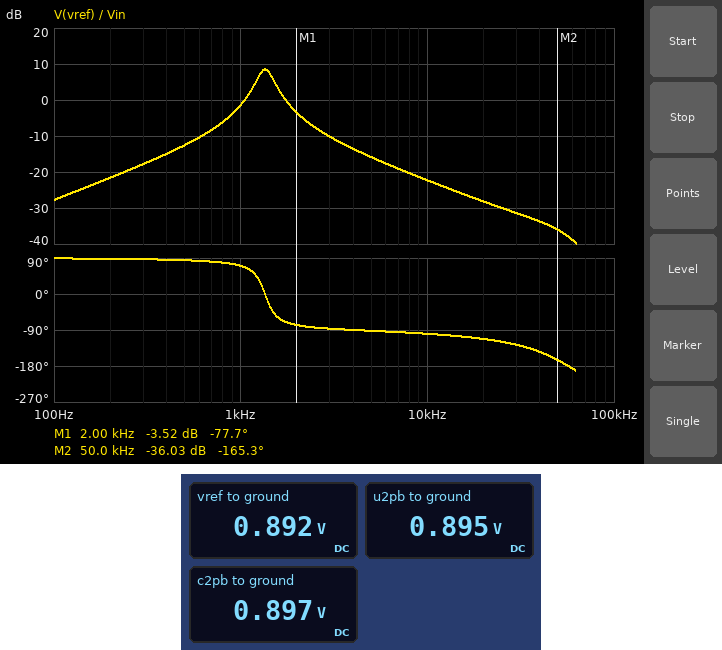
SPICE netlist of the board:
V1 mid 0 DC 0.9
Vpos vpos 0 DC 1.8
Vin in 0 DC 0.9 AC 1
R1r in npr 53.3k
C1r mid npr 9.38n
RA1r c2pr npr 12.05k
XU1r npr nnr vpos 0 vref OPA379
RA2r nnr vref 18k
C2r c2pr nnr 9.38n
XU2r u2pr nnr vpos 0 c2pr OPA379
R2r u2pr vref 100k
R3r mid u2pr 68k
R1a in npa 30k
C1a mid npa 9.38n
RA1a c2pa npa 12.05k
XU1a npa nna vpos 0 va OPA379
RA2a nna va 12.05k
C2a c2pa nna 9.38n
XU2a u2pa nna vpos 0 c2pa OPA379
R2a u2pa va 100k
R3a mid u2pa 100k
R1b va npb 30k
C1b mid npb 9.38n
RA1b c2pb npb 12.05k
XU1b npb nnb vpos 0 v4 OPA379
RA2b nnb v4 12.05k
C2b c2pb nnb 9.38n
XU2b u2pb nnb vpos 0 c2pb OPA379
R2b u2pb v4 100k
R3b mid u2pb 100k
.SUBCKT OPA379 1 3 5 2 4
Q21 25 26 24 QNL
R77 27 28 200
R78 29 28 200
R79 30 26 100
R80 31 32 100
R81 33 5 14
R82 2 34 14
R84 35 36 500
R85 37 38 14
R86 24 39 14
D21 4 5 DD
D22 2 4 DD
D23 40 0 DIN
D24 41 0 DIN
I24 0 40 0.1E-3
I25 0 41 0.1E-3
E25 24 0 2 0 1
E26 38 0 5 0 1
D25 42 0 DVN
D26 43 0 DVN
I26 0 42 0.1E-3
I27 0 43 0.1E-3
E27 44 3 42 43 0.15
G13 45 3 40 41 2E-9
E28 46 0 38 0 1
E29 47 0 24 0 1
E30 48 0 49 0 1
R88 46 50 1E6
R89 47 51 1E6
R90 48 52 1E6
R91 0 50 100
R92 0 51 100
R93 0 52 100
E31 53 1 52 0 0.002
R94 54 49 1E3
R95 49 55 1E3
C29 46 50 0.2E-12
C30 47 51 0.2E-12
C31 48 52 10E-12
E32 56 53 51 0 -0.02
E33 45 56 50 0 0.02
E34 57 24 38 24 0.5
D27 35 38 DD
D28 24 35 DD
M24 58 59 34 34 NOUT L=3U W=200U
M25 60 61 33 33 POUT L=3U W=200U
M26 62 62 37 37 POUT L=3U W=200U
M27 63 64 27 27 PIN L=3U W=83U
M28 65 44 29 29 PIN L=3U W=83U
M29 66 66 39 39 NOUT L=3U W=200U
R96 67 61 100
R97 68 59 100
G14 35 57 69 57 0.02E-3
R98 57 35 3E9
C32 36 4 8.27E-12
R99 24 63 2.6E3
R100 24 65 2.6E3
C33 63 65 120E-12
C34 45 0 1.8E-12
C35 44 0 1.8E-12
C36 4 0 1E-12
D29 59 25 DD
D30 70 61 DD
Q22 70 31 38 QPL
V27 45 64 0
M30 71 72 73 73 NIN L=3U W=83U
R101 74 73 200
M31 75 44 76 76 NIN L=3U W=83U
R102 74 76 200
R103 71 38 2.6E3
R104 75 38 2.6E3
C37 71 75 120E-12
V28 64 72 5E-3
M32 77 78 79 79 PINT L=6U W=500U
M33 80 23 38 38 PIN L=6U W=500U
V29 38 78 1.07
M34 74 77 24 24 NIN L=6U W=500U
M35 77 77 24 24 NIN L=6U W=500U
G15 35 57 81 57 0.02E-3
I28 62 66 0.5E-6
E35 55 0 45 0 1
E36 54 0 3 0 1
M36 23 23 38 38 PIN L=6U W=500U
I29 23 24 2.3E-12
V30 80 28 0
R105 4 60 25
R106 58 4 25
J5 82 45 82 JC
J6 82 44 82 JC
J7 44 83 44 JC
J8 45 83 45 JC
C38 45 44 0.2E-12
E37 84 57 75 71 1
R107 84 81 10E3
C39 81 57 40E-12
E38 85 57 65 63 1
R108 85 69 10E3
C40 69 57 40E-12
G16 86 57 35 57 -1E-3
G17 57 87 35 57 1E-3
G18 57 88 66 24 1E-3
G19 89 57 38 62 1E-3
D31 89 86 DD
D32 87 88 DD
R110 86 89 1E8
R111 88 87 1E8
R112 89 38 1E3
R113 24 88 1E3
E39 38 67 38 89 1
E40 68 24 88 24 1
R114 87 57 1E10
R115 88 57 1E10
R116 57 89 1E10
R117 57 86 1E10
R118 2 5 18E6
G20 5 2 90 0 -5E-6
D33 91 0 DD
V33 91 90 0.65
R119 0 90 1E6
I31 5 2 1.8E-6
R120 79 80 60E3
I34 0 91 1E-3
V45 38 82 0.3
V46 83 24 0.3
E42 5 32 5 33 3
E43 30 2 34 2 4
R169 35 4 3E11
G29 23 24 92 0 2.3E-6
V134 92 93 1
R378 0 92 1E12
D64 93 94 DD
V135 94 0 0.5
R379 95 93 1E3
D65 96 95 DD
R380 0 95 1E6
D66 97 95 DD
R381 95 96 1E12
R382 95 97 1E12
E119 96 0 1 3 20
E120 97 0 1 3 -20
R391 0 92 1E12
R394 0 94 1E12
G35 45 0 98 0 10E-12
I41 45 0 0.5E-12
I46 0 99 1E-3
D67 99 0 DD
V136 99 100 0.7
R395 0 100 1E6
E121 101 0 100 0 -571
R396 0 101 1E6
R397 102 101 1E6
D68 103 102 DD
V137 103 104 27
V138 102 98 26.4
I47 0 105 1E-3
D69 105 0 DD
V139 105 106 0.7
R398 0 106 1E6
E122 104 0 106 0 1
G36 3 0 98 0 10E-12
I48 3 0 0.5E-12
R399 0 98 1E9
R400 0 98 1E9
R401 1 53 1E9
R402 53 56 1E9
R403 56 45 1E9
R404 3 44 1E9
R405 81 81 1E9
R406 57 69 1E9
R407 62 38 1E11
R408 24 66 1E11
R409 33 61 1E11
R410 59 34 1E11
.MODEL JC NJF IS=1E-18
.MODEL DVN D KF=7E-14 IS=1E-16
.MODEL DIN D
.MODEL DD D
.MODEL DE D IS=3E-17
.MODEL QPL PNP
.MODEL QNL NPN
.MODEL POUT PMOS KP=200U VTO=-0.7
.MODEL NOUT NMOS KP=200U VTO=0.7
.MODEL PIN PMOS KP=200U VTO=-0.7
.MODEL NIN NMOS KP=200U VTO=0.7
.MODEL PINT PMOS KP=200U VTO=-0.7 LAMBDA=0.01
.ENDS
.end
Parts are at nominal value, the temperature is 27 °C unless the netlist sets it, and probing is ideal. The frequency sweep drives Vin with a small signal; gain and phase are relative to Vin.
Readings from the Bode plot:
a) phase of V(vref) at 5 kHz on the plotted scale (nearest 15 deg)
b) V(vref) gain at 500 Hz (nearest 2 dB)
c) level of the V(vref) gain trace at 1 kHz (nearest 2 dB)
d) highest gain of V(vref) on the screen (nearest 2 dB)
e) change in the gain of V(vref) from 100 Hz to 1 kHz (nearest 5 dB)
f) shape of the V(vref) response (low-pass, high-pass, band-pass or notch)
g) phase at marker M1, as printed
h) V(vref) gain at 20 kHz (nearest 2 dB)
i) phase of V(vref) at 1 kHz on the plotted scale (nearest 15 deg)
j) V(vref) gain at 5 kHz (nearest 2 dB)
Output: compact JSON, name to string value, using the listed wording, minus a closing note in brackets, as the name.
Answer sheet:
{"phase of V(vref) at 5 kHz on the plotted scale": "-90 deg", "V(vref) gain at 500 Hz": "-12 dB", "level of the V(vref) gain trace at 1 kHz": "-2 dB", "highest gain of V(vref) on the screen": "8 dB", "change in the gain of V(vref) from 100 Hz to 1 kHz": "25 dB", "shape of the V(vref) response": "band-pass", "phase at marker M1, as printed": "-77.7 deg", "V(vref) gain at 20 kHz": "-28 dB", "phase of V(vref) at 1 kHz on the plotted scale": "75 deg", "V(vref) gain at 5 kHz": "-16 dB"}
